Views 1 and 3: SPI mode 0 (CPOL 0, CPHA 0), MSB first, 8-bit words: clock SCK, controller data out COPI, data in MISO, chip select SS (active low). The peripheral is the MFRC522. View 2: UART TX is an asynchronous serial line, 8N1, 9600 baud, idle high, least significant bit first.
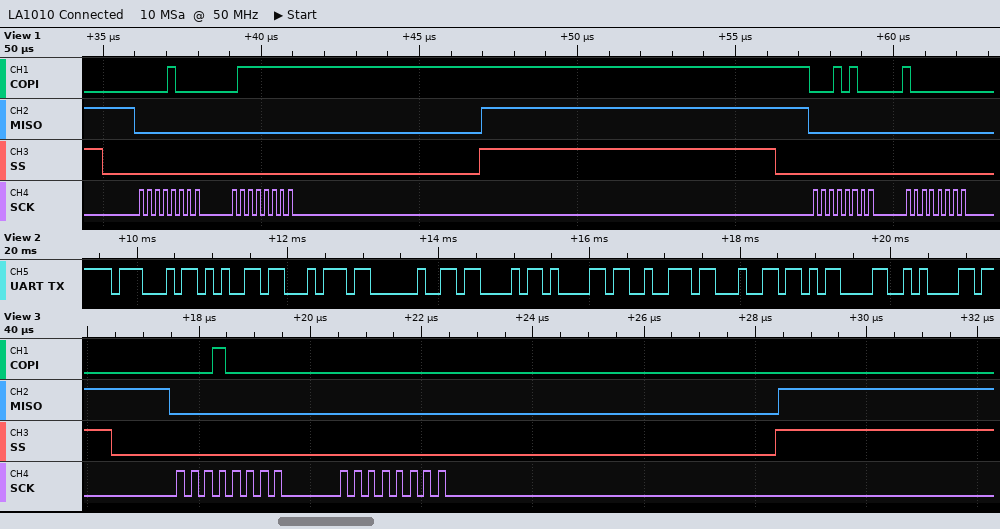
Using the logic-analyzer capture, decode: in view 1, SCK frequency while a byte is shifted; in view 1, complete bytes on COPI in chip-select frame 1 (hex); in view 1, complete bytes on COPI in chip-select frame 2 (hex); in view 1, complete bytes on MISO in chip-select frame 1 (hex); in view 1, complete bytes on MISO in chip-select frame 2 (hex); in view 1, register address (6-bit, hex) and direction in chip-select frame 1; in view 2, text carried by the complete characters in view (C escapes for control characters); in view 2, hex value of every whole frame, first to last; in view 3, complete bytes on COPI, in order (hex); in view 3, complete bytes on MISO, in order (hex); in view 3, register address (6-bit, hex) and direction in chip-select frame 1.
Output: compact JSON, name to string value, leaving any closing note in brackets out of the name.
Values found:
{"in view 1, SCK frequency while a byte is shifted": "4 MHz", "in view 1, complete bytes on COPI in chip-select frame 1": "08 7F", "in view 1, complete bytes on COPI in chip-select frame 2": "14 80", "in view 1, complete bytes on MISO in chip-select frame 1": "00 00", "in view 1, complete bytes on MISO in chip-select frame 2": "00 00", "in view 1, register address (6-bit, hex) and direction in chip-select frame 1": "0x04 write", "in view 2, text carried by the complete characters in view": "\"Get Card\\r\\n\"", "in view 2, hex value of every whole frame, first to last": "0x47 0x65 0x74 0x20 0x43 0x61 0x72 0x64 0x0D 0x0A", "in view 3, complete bytes on COPI, in order": "0x10 0x00", "in view 3, complete bytes on MISO, in order": "0x00 0x00", "in view 3, register address (6-bit, hex) and direction in chip-select frame 1": "0x08 write"}
